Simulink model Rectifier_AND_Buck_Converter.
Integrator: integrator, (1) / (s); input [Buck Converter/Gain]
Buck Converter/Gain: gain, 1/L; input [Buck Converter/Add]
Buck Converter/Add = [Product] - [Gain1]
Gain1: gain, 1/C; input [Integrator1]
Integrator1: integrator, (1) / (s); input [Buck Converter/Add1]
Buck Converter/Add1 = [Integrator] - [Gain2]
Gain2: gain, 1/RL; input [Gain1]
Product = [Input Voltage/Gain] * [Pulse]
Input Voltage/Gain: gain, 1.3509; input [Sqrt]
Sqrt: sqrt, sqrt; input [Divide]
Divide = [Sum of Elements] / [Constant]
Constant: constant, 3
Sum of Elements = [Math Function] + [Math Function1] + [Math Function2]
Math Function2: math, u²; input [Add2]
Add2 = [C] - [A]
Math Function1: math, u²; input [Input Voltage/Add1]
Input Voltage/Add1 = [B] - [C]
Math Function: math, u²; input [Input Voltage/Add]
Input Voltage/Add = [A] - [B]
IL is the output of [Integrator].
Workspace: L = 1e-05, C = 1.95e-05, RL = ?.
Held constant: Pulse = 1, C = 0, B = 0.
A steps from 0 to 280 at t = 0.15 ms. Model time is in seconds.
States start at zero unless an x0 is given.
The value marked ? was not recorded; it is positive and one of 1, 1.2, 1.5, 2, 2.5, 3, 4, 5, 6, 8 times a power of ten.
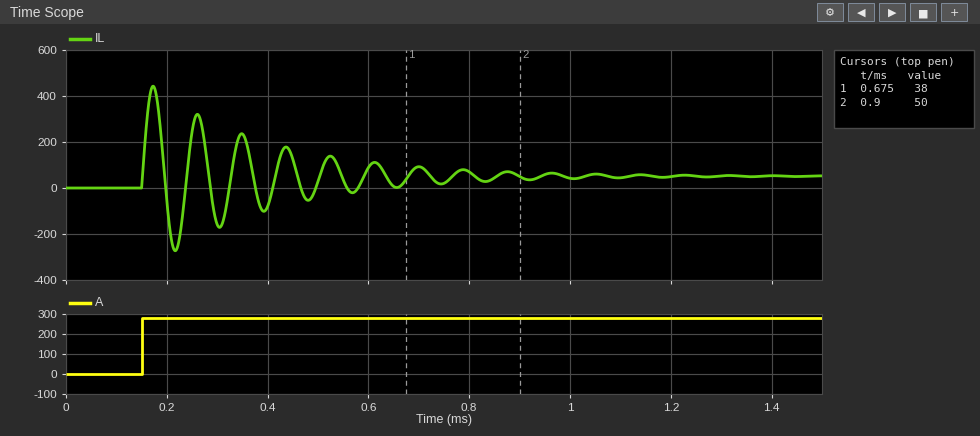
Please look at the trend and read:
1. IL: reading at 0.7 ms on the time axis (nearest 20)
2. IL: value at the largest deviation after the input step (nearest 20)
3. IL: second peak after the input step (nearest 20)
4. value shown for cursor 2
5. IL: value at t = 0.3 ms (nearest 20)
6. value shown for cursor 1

100
440
320
50
-160
38
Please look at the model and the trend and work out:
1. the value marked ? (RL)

6
